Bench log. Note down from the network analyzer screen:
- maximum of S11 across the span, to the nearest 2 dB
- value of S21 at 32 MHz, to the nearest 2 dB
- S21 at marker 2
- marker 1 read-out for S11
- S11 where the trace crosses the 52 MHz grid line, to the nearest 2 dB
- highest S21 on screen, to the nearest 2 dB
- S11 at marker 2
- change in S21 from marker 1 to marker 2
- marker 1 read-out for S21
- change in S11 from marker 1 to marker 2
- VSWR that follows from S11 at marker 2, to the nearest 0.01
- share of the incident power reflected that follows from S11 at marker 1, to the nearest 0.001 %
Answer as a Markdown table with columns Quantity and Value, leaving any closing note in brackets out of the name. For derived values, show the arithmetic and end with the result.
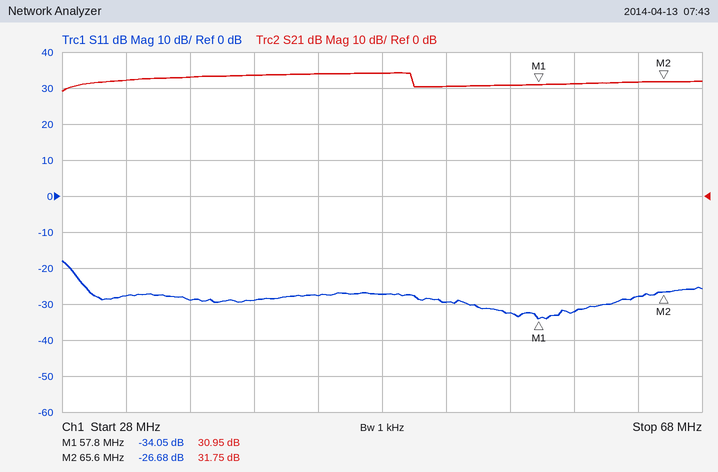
| Quantity | Value |
|---|---|
| maximum of S11 across the span, to the nearest 2 dB | -18 dB |
| value of S21 at 32 MHz, to the nearest 2 dB | 32 dB |
| S21 at marker 2 | 31.75 dB |
| marker 1 read-out for S11 | -34.05 dB |
| S11 where the trace crosses the 52 MHz grid line, to the nearest 2 dB | -30 dB |
| highest S21 on screen, to the nearest 2 dB | 34 dB |
| S11 at marker 2 | -26.68 dB |
| change in S21 from marker 1 to marker 2 | 31.75 − (30.95) = 0.80 dB |
| marker 1 read-out for S21 | 30.95 dB |
| change in S11 from marker 1 to marker 2 | -26.68 − (-34.05) = 7.37 dB |
| VSWR that follows from S11 at marker 2, to the nearest 0.01 | (1 + 0.0463)/(1 − 0.0463) ≈ 1.10 |
| share of the incident power reflected that follows from S11 at marker 1, to the nearest 0.001 % | 10^(-34.05/10) ≈ 0.039 % |
